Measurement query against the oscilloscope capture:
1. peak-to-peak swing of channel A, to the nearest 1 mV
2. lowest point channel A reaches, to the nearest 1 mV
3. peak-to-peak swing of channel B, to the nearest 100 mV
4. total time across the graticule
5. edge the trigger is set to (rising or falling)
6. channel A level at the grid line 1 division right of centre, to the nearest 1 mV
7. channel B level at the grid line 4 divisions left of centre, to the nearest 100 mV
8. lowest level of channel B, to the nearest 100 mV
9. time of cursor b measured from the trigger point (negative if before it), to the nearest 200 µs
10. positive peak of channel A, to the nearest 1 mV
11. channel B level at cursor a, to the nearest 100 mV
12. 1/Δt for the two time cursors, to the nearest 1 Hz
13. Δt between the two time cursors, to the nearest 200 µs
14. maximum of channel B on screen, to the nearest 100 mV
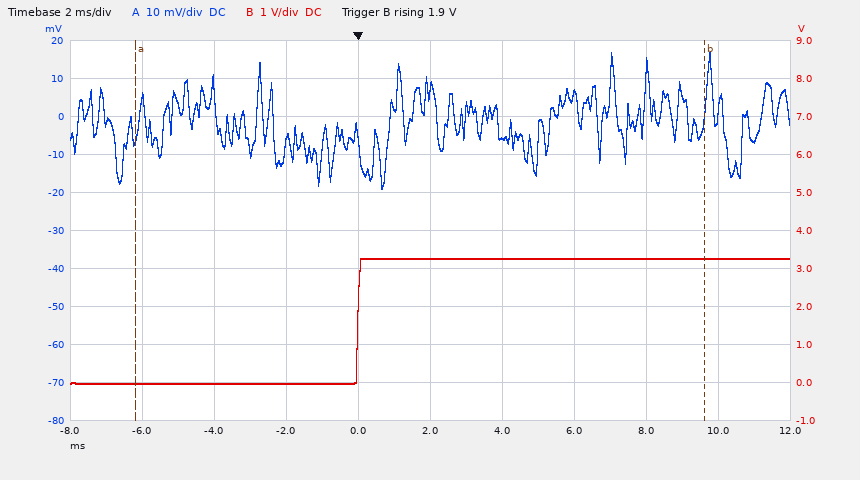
36 mV
-19 mV
3.3 V
20 ms
rising
-6 mV
0.0 V
0.0 V
+9.6 ms
17 mV
0.0 V
63 Hz
15.8 ms
3.3 V
